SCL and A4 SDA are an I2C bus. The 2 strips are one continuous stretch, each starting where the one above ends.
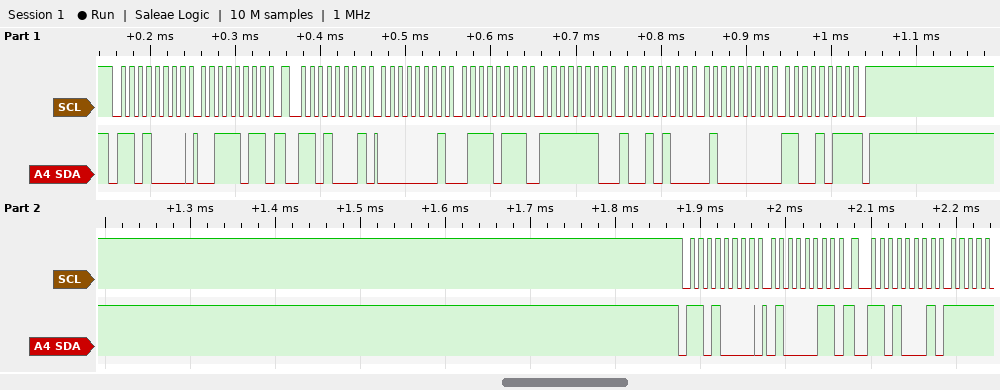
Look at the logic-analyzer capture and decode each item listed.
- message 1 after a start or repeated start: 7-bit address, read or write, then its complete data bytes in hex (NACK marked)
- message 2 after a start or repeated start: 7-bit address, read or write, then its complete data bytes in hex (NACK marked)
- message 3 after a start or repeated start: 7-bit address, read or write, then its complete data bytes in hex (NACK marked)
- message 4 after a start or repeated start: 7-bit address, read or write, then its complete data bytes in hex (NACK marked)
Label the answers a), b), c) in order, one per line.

a) 0x68 write: 3B
b) 0x68 read: 01 77 FE 94 40 CB NACK
c) 0x68 write: 43
d) 0x68 read
